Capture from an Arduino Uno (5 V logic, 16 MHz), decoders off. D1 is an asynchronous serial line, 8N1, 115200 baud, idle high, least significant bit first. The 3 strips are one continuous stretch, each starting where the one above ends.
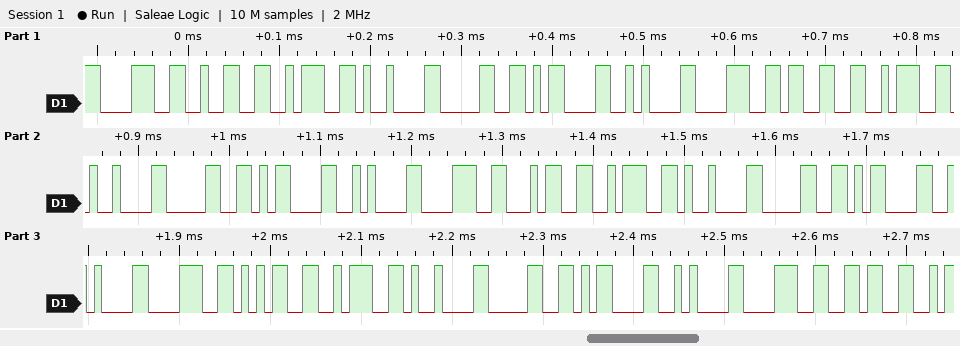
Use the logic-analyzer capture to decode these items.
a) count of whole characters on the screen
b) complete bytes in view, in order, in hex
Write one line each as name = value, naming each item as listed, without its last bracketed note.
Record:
count of whole characters on the screen = 30
complete bytes in view, in order, in hex = 38 32 3A 09 30 0D 0A 38 33 3A 09 30 0D 0A 38 34 3A 09 30 0D 0A 38 35 3A 09 30 0D 0A 38 36
